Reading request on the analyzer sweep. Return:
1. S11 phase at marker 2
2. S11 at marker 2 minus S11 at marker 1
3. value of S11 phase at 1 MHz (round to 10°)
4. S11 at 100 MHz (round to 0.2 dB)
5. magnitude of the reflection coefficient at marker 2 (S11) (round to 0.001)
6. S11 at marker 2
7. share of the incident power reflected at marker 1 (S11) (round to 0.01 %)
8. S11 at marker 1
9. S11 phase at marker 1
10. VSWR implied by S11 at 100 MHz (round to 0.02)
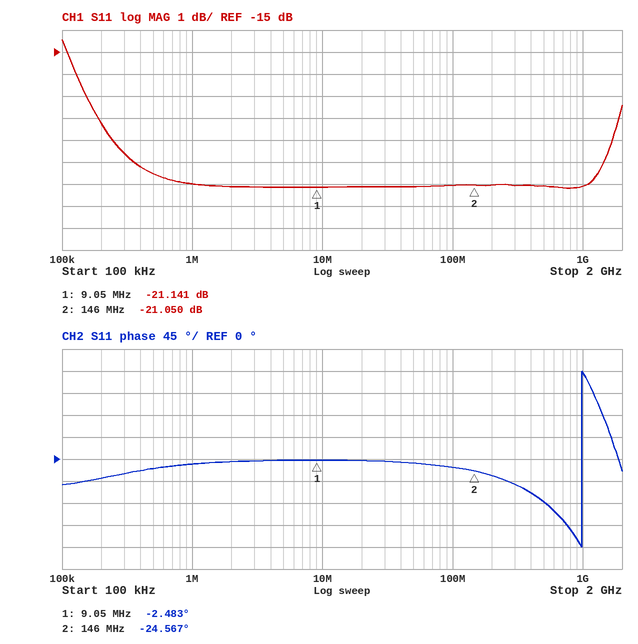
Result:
-24.567°
0.091 dB
-10°
-21.0 dB
0.089
-21.050 dB
0.77 %
-21.141 dB
-2.483°
1.20
